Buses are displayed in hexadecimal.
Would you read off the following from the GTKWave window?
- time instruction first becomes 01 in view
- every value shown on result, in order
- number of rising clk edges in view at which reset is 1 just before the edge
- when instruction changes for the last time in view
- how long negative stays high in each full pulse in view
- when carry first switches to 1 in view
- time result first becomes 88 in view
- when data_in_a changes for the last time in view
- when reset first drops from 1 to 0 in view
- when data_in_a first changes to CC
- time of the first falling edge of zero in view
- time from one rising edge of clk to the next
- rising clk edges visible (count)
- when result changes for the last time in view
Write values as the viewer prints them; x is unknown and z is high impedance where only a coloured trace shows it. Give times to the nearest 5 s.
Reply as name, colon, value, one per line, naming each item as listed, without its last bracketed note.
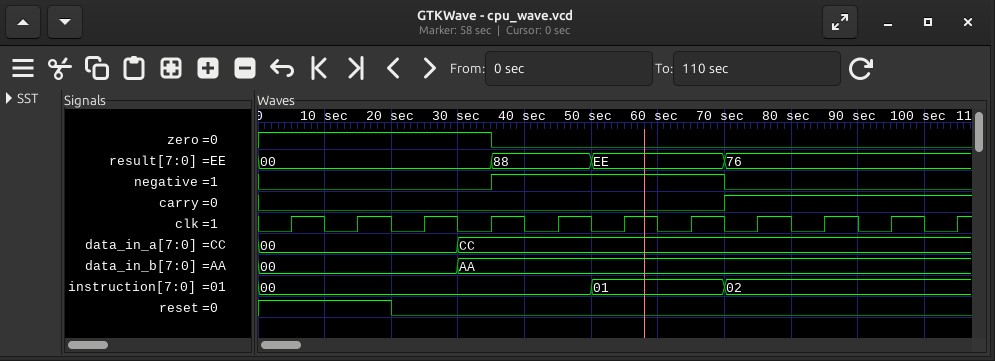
time instruction first becomes 01 in view: 50 s
every value shown on result, in order: 00, 88, EE, 76
number of rising clk edges in view at which reset is 1 just before the edge: 2
when instruction changes for the last time in view: 70 s
how long negative stays high in each full pulse in view: 35 s
when carry first switches to 1 in view: 70 s
time result first becomes 88 in view: 35 s
when data_in_a changes for the last time in view: 30 s
when reset first drops from 1 to 0 in view: 20 s
when data_in_a first changes to CC: 30 s
time of the first falling edge of zero in view: 35 s
time from one rising edge of clk to the next: 10 s
rising clk edges visible: 11
when result changes for the last time in view: 70 s
